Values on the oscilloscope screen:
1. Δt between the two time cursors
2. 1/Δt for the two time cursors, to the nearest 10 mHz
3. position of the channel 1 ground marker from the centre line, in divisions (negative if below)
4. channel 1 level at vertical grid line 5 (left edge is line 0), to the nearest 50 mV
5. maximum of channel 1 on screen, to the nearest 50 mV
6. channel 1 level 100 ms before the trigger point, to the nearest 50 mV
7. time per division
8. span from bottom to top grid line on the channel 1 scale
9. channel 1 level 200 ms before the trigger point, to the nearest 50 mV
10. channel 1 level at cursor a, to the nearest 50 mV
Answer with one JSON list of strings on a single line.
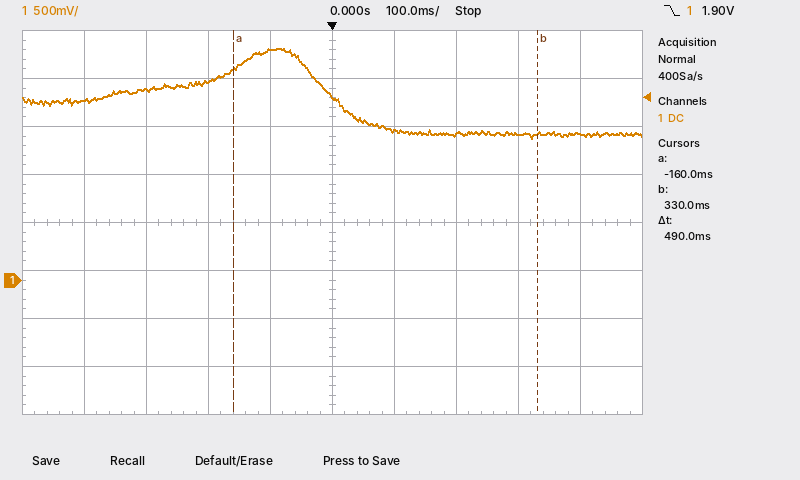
["490 ms", "2.04 Hz", "-1.2 div", "1.90 V", "2.40 V", "2.40 V", "100 ms", "4 V", "2.05 V", "2.20 V"]
